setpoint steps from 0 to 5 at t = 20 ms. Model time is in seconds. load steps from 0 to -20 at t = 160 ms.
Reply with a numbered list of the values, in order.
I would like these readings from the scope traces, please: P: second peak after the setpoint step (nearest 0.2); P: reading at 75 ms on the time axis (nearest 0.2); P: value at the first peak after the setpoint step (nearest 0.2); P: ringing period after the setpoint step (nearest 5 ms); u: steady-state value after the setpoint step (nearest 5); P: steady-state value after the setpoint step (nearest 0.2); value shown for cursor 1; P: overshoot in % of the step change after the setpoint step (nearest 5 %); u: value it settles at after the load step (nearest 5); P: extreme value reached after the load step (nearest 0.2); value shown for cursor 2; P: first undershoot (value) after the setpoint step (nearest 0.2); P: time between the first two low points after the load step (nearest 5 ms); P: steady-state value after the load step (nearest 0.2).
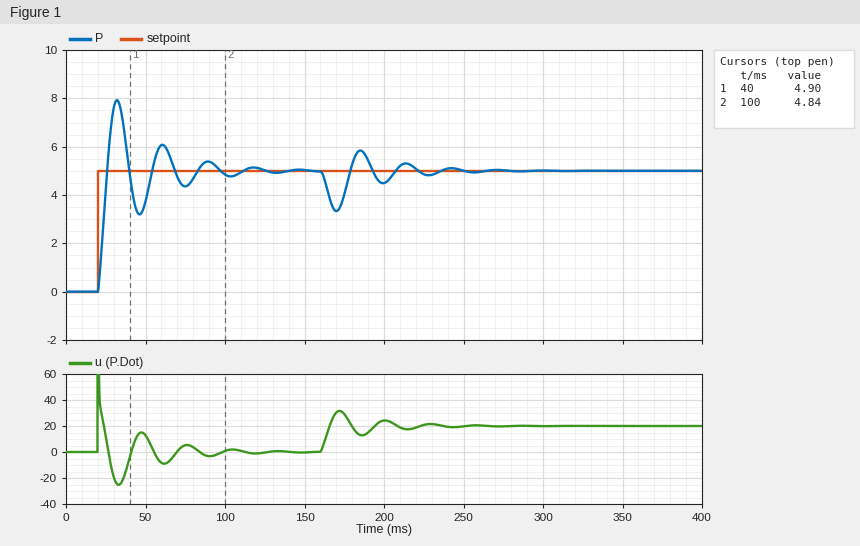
1. 6.0
2. 4.4
3. 8.0
4. 30 ms
5. 0
6. 5.0
7. 4.90
8. 60 %
9. 20
10. 3.4
11. 4.84
12. 3.2
13. 30 ms
14. 5.0
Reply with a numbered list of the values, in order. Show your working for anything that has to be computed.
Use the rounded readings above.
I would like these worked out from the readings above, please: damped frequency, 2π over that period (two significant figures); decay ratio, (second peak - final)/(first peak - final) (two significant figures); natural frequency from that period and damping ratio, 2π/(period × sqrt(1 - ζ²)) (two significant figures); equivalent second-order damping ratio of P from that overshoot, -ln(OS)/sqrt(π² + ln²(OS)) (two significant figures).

1. 2π / 30 = 0.21 rad/ms
2. (6 - 5) / (8 - 5) = 0.33
3. 2π / (30 × sqrt(1 - 0.16²)) = 0.21 rad/ms
4. ln(0.6) = -0.511; 0.511 / sqrt(9.870 + 0.261) = 0.16
